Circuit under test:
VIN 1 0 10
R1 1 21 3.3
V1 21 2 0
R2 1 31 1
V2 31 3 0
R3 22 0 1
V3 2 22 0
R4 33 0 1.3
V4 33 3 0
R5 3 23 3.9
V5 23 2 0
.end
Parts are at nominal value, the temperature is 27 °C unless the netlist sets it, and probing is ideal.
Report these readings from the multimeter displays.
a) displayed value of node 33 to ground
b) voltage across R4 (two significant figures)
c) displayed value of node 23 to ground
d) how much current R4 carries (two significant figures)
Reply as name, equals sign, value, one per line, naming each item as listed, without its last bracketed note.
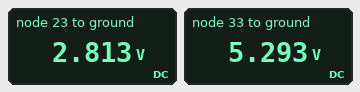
displayed value of node 33 to ground = 5.293 V
voltage across R4 = 5.3 V
displayed value of node 23 to ground = 2.813 V
how much current R4 carries = 4.1 A
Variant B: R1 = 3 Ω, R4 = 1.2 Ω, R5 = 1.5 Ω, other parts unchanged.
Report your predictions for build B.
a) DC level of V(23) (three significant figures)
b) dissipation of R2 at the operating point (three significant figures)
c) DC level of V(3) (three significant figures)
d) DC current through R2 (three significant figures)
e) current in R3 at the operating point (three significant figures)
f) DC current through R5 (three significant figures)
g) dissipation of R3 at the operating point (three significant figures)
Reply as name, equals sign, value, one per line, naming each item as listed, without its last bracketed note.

DC level of V(23) = 3.29 V
dissipation of R2 at the operating point = 26.2 W
DC level of V(3) = 4.88 V
DC current through R2 = 5.12 A
current in R3 at the operating point = 3.29 A
DC current through R5 = 1.06 A
dissipation of R3 at the operating point = 10.8 W
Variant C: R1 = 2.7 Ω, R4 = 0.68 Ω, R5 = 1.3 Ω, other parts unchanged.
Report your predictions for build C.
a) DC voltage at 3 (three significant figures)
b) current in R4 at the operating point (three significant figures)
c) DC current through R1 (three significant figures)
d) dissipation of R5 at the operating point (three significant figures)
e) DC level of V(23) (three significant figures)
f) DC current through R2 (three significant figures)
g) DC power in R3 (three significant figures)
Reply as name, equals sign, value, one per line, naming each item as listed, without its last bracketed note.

DC voltage at 3 = 3.82 V
current in R4 at the operating point = 5.62 A
DC current through R1 = 2.55 A
dissipation of R5 at the operating point = 397 mW
DC level of V(23) = 3.11 V
DC current through R2 = 6.18 A
DC power in R3 = 9.65 W
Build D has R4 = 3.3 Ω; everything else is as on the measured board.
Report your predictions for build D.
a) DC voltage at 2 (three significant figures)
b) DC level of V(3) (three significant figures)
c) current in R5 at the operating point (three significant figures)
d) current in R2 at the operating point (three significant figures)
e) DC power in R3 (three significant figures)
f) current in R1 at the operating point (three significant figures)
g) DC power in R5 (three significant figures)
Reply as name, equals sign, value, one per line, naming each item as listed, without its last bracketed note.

DC voltage at 2 = 3.08 V
DC level of V(3) = 6.92 V
current in R5 at the operating point = 984 mA
current in R2 at the operating point = 3.08 A
DC power in R3 = 9.49 W
current in R1 at the operating point = 2.10 A
DC power in R5 = 3.78 W
